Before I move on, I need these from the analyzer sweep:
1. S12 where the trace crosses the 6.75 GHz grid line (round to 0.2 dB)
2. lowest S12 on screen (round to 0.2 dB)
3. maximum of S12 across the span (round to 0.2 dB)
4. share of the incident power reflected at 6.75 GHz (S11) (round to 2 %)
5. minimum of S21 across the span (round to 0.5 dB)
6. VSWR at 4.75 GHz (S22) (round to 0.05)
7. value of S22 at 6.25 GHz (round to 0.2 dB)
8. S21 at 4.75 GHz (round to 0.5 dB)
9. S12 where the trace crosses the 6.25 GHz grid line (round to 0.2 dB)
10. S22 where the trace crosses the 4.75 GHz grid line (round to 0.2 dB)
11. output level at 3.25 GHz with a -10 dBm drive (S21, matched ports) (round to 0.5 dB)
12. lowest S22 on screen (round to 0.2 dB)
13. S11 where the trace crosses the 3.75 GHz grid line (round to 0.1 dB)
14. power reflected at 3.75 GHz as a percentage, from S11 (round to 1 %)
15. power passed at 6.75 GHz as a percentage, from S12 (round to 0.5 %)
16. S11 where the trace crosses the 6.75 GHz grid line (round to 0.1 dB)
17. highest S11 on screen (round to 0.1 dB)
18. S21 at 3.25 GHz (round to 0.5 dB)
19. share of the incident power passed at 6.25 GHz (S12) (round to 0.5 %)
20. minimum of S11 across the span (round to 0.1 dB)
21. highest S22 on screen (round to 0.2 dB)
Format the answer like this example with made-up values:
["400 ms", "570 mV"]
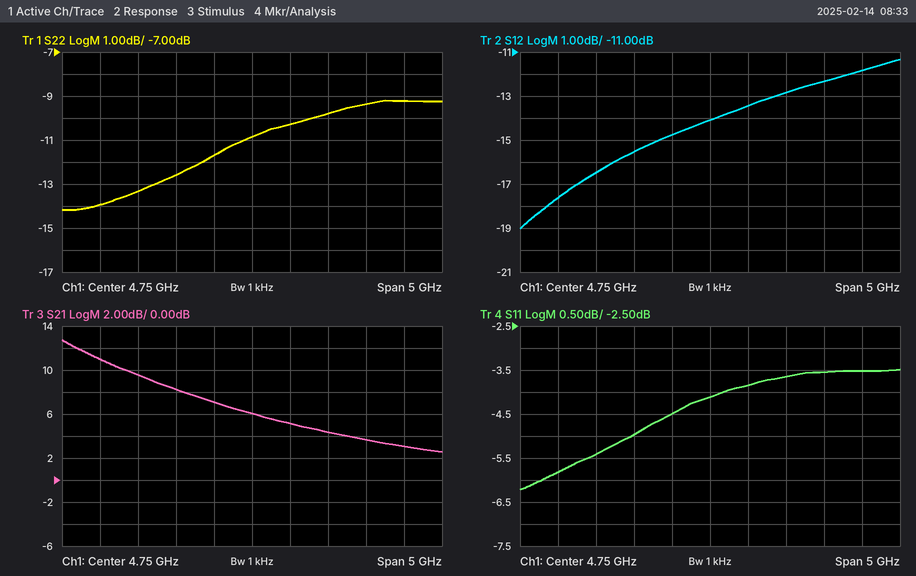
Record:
["-11.8 dB", "-19.0 dB", "-11.4 dB", "44 %", "2.5 dB", "1.80", "-9.4 dB", "6.0 dB", "-12.4 dB", "-10.8 dB", "-0.5 dBm", "-14.2 dB", "-5.0 dB", "32 %", "6.5 %", "-3.5 dB", "-3.5 dB", "9.5 dB", "6.0 %", "-6.2 dB", "-9.2 dB"]
